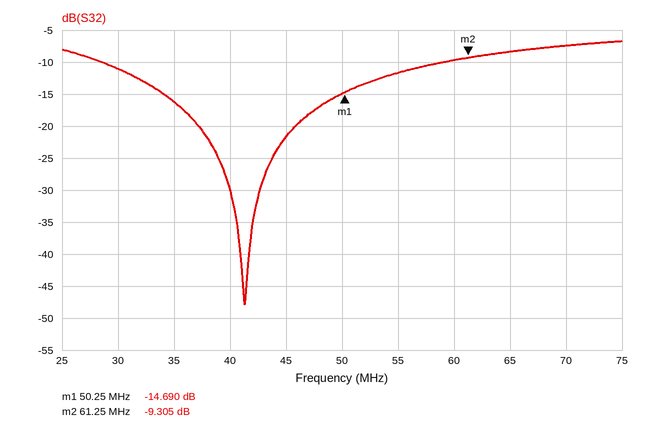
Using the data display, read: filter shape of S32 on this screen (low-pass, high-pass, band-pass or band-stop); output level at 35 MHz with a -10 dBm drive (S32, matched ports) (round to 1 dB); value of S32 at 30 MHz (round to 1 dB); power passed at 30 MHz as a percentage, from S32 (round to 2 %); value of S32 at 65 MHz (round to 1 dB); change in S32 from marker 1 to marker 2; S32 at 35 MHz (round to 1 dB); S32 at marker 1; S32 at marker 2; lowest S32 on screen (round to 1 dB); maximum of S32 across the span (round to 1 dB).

band-stop
-26 dBm
-11 dB
8 %
-8 dB
5.385 dB
-16 dB
-14.690 dB
-9.305 dB
-48 dB
-7 dB
